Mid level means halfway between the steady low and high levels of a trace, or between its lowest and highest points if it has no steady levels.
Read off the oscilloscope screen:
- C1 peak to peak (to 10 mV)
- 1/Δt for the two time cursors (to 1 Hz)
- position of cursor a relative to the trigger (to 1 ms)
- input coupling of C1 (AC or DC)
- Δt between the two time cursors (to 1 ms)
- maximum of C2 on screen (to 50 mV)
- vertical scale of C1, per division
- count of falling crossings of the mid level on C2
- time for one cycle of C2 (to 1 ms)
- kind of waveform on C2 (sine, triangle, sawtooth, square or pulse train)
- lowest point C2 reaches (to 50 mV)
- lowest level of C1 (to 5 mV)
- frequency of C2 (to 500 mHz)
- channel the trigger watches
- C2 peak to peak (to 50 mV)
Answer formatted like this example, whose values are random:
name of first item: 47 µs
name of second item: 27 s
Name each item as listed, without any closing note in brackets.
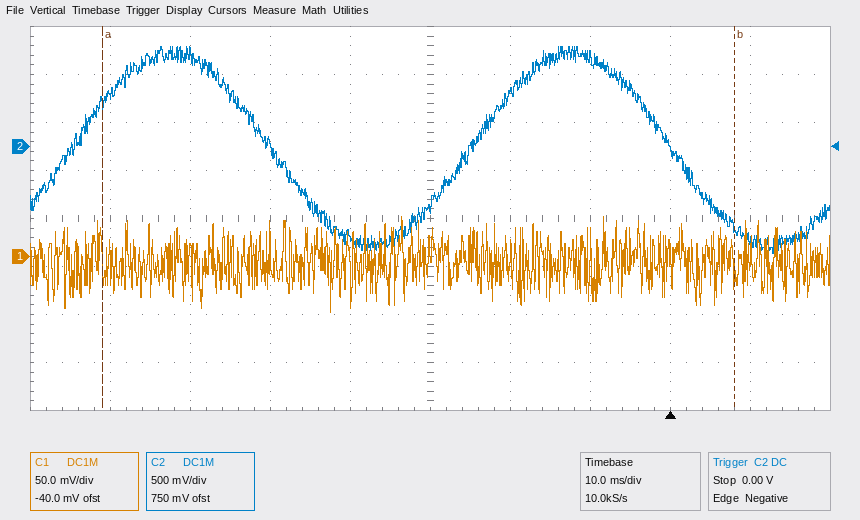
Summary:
C1 peak to peak: 100 mV
1/Δt for the two time cursors: 13 Hz
position of cursor a relative to the trigger: -71 ms
input coupling of C1: DC
Δt between the two time cursors: 79 ms
maximum of C2 on screen: 1.05 V
vertical scale of C1, per division: 50 mV
count of falling crossings of the mid level on C2: 2
time for one cycle of C2: 50 ms
kind of waveform on C2: sine
lowest point C2 reaches: -1.10 V
lowest level of C1: -60 mV
frequency of C2: 20.0 Hz
channel the trigger watches: C2
C2 peak to peak: 2.15 V
